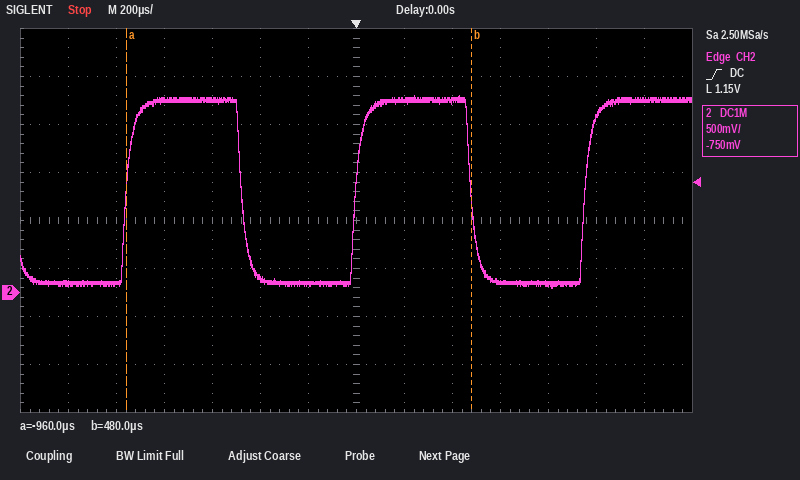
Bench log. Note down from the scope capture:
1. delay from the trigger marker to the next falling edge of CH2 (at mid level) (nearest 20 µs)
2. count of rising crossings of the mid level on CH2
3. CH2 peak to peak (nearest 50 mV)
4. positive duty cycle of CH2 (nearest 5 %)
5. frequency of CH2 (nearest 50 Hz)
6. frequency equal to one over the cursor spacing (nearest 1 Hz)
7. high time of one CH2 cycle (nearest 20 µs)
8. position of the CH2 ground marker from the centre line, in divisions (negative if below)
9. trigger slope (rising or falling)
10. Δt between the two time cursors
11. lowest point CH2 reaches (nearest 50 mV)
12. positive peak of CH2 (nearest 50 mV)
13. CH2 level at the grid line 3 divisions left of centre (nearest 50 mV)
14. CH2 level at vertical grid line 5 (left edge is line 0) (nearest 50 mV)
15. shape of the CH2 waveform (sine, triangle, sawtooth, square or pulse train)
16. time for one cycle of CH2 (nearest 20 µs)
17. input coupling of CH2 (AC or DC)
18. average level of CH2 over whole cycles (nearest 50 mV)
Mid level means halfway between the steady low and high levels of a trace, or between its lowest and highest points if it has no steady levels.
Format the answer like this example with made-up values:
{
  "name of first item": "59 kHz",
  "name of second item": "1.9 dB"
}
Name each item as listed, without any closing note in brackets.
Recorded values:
{
  "delay from the trigger marker to the next falling edge of CH2 (at mid level)": "480 µs",
  "count of rising crossings of the mid level on CH2": "3",
  "CH2 peak to peak": "2.00 V",
  "positive duty cycle of CH2": "50 %",
  "frequency of CH2": "1.05 kHz",
  "frequency equal to one over the cursor spacing": "694 Hz",
  "high time of one CH2 cycle": "480 µs",
  "position of the CH2 ground marker from the centre line, in divisions": "-1.5 div",
  "trigger slope": "rising",
  "Δt between the two time cursors": "1.44 ms",
  "lowest point CH2 reaches": "50 mV",
  "positive peak of CH2": "2.05 V",
  "CH2 level at the grid line 3 divisions left of centre": "2.00 V",
  "CH2 level at vertical grid line 5 (left edge is line 0)": "150 mV",
  "shape of the CH2 waveform": "square",
  "time for one cycle of CH2": "960 µs",
  "input coupling of CH2": "DC",
  "average level of CH2 over whole cycles": "1.05 V"
}
